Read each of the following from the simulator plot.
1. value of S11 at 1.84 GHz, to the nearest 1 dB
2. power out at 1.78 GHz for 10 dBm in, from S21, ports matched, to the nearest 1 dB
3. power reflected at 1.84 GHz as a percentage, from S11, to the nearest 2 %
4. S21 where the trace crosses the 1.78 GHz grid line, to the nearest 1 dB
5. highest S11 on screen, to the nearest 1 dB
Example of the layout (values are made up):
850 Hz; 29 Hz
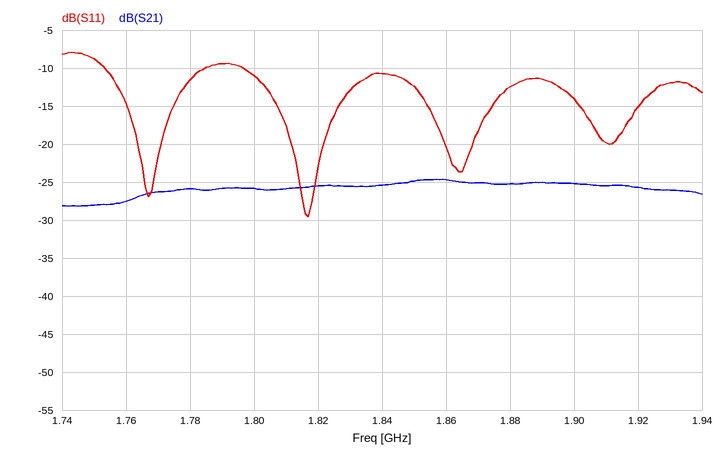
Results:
-11 dB; -16 dBm; 8 %; -26 dB; -8 dB
